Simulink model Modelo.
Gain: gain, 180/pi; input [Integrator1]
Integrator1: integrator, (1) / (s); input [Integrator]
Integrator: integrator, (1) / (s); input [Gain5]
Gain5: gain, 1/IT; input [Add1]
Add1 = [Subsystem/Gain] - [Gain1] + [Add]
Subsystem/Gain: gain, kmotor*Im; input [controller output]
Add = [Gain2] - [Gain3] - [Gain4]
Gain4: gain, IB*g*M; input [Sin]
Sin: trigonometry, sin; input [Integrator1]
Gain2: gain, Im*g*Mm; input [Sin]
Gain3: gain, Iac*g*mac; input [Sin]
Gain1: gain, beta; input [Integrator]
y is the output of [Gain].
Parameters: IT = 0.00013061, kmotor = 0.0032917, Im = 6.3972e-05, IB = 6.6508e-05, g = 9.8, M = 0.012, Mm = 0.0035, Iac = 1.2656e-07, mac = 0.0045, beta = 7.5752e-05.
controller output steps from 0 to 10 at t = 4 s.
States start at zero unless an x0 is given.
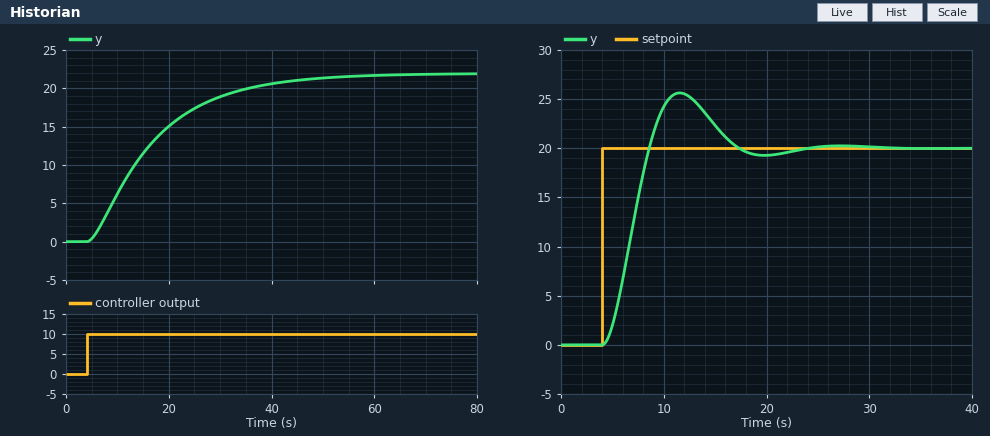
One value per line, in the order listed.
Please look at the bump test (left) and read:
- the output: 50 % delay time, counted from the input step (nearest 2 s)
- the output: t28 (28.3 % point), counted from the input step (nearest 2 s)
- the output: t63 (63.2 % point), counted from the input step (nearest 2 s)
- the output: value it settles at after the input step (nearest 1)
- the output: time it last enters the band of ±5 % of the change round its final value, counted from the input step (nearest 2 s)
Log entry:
10 s
6 s
14 s
22
38 s
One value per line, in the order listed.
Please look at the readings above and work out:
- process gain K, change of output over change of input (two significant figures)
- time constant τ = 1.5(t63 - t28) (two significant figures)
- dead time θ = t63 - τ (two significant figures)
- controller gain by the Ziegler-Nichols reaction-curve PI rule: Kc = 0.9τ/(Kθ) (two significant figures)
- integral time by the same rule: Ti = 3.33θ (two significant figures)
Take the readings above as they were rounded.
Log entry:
2.2
12 s
2.0 s
2.5
6.7 s
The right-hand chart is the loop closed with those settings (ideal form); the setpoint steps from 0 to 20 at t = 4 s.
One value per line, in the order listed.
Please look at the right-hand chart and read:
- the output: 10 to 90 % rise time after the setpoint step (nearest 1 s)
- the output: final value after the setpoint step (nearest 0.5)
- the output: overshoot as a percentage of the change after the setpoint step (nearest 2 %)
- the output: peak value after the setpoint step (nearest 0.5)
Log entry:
3 s
20.0
28 %
25.5
